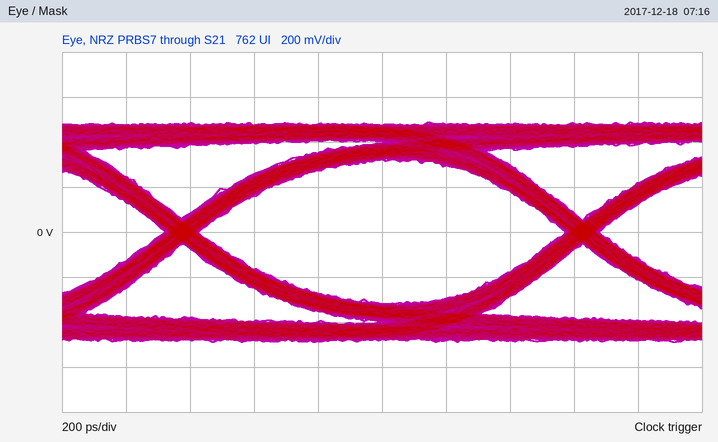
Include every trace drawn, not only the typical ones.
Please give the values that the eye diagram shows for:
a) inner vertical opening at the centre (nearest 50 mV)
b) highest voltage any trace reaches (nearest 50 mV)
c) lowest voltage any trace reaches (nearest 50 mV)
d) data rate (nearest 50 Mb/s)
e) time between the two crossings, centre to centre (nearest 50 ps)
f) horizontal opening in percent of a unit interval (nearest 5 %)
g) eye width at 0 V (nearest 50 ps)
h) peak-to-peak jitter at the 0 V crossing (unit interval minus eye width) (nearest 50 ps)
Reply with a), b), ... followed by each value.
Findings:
a) 650 mV
b) 500 mV
c) -500 mV
d) 800 Mb/s
e) 1.25 ns
f) 90 %
g) 1.15 ns
h) 100 ps
